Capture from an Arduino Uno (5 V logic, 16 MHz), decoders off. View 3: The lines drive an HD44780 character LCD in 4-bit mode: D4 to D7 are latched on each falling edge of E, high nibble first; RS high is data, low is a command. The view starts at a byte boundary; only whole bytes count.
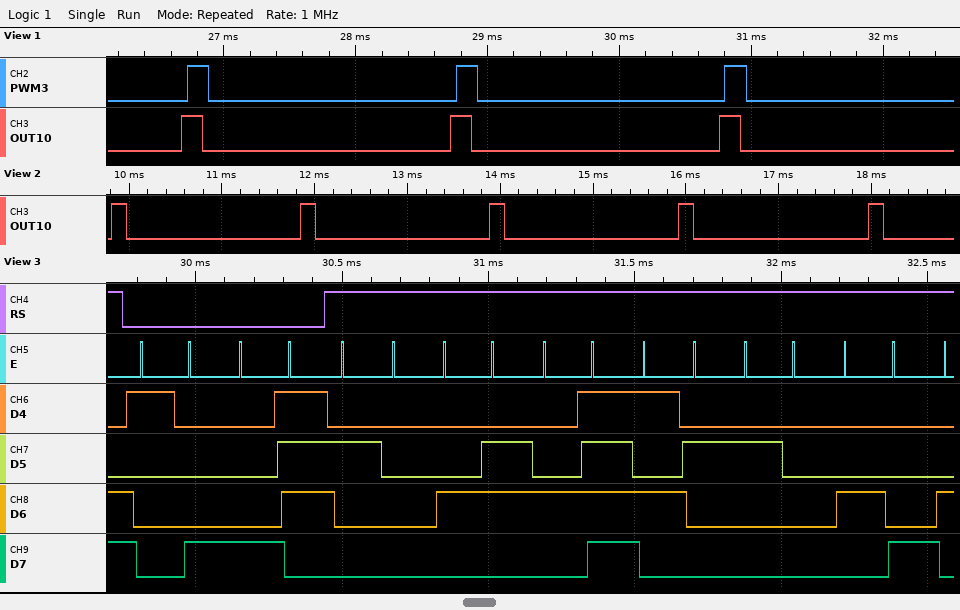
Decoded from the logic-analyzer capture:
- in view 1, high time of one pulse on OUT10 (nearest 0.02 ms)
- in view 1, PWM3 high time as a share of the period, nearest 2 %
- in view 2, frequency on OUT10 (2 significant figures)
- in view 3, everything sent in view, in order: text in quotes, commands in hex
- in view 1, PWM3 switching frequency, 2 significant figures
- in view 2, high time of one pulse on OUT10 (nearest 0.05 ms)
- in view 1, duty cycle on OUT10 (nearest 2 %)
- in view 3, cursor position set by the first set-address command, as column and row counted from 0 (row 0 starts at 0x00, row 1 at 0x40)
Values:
0.16 ms
8 %
490 Hz
0x18 0x87 " FOR H"
490 Hz
0.15 ms
8 %
column 7, row 0
